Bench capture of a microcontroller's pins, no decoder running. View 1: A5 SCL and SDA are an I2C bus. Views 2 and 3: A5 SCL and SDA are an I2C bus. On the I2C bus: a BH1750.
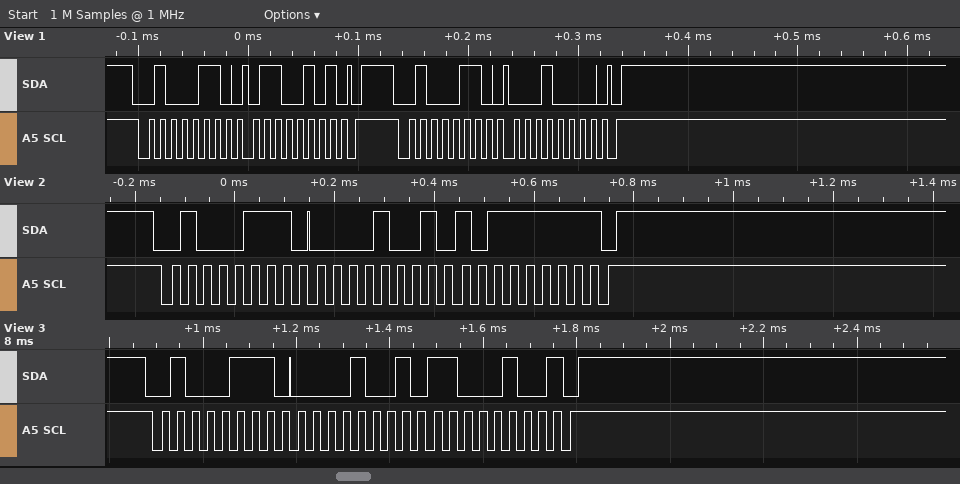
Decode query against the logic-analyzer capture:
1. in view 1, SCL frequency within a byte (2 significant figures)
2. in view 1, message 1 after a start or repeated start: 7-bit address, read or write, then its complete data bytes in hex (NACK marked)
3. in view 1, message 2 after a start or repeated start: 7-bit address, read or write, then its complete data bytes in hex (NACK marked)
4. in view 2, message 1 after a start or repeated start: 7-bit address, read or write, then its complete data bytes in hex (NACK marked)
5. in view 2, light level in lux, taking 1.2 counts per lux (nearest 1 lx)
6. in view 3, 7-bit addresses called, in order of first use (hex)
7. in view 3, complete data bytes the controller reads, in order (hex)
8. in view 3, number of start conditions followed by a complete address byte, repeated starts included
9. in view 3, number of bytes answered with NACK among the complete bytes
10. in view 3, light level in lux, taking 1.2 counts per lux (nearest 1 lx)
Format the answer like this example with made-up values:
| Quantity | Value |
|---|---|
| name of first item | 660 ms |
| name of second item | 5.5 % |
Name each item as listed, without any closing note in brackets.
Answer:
| Quantity | Value |
|---|---|
| in view 1, SCL frequency within a byte | 100 kHz |
| in view 1, message 1 after a start or repeated start: 7-bit address, read or write, then its complete data bytes in hex | 0x23 write: 65 |
| in view 1, message 2 after a start or repeated start: 7-bit address, read or write, then its complete data bytes in hex | 0x23 write: 10 |
| in view 2, message 1 after a start or repeated start: 7-bit address, read or write, then its complete data bytes in hex | 0x23 read: 09 BF NACK |
| in view 2, light level in lux, taking 1.2 counts per lux | 2079 lx |
| in view 3, 7-bit addresses called, in order of first use | 0x23 |
| in view 3, complete data bytes the controller reads, in order | 09 C4 |
| in view 3, number of start conditions followed by a complete address byte, repeated starts included | 1 |
| in view 3, number of bytes answered with NACK among the complete bytes | 1 |
| in view 3, light level in lux, taking 1.2 counts per lux | 2083 lx |
